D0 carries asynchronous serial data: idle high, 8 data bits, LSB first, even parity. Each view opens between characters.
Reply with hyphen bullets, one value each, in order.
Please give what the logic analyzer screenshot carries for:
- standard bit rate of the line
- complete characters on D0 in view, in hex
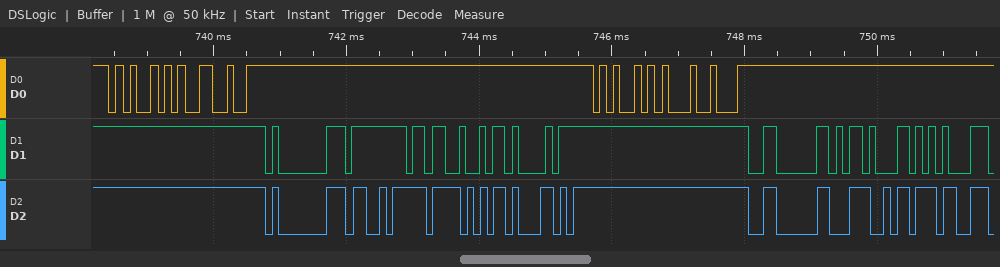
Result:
- 9600 baud
- A5, 26, A5, 24
